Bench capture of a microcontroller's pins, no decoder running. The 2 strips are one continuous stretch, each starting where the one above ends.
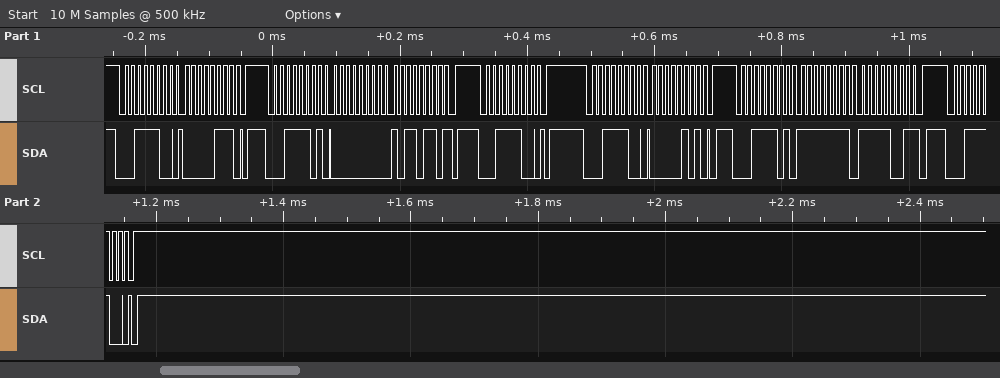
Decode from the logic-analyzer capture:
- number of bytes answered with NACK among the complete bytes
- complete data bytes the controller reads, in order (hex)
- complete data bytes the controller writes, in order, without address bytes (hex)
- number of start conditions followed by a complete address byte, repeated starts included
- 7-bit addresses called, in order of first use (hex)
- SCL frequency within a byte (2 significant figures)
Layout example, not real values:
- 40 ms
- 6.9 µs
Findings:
- 2
- 00 B6 FF F9
- 07 05
- 6
- 0x1E
- 100 kHz
